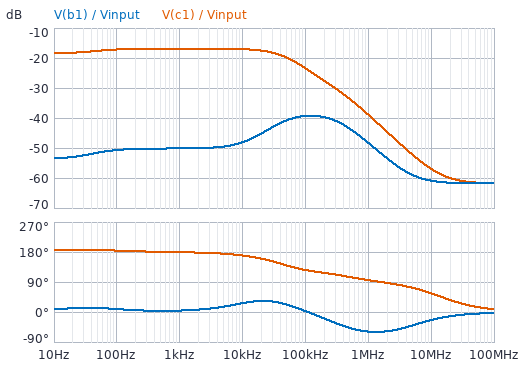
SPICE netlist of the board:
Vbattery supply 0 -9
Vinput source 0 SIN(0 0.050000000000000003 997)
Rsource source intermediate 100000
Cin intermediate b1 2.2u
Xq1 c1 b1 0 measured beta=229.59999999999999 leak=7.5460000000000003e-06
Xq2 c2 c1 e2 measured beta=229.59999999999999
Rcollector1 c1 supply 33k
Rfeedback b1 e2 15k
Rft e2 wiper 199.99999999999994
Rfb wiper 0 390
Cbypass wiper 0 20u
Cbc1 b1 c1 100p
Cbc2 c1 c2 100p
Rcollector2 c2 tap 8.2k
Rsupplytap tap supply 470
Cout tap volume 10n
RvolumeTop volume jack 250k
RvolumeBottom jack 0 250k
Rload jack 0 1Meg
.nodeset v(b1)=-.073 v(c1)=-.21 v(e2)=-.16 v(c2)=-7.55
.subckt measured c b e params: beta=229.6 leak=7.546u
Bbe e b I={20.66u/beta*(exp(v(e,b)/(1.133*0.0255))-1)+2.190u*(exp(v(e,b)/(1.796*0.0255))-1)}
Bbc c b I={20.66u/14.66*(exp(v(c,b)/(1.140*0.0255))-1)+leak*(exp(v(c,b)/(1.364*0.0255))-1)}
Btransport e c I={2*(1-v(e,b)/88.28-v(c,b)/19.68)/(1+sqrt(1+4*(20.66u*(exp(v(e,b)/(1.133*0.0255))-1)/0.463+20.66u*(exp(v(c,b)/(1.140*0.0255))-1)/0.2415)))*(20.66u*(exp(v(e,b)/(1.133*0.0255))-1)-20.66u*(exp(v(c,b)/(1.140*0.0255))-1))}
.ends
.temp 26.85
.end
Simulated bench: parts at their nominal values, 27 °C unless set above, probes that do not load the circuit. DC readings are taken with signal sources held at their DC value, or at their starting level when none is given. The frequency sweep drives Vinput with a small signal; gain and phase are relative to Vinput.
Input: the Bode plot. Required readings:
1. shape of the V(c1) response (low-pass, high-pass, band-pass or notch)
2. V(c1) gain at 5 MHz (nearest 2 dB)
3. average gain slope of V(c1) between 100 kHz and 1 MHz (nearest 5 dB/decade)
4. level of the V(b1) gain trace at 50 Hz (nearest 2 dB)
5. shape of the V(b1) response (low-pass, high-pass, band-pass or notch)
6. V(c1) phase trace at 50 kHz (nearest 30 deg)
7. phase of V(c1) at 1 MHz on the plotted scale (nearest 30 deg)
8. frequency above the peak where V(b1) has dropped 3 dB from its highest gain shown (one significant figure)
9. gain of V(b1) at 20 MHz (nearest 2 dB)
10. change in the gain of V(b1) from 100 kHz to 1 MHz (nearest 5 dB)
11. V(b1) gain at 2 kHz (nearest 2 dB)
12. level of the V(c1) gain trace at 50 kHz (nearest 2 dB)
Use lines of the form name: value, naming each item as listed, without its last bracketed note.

shape of the V(c1) response: low-pass
V(c1) gain at 5 MHz: -52 dB
average gain slope of V(c1) between 100 kHz and 1 MHz: -15 dB/decade
level of the V(b1) gain trace at 50 Hz: -52 dB
shape of the V(b1) response: band-pass
V(c1) phase trace at 50 kHz: 150 deg
phase of V(c1) at 1 MHz on the plotted scale: 90 deg
frequency above the peak where V(b1) has dropped 3 dB from its highest gain shown: 400 kHz
gain of V(b1) at 20 MHz: -62 dB
change in the gain of V(b1) from 100 kHz to 1 MHz: -10 dB
V(b1) gain at 2 kHz: -50 dB
level of the V(c1) gain trace at 50 kHz: -20 dB
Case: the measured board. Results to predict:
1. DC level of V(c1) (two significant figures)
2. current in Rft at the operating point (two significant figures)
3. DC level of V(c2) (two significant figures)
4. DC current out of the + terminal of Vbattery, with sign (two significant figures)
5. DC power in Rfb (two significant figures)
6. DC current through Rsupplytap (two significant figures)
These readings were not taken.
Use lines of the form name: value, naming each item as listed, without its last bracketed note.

DC level of V(c1): -150 mV
current in Rft at the operating point: 170 µA
DC level of V(c2): -7.5 V
DC current out of the + terminal of Vbattery, with sign: -440 µA
DC power in Rfb: 11 µW
DC current through Rsupplytap: 180 µA
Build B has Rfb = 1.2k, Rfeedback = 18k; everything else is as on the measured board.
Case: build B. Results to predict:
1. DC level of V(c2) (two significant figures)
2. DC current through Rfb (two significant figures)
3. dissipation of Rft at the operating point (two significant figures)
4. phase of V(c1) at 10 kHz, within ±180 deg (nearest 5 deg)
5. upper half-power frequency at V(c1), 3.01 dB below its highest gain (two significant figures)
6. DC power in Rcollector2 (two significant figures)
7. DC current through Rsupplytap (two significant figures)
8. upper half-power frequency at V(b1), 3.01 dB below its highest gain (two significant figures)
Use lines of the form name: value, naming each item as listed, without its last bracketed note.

DC level of V(c2): -8.2 V
DC current through Rfb: 81 µA
dissipation of Rft at the operating point: 1.3 µW
phase of V(c1) at 10 kHz, within ±180 deg: 170 deg
upper half-power frequency at V(c1), 3.01 dB below its highest gain: 55 kHz
DC power in Rcollector2: 66 µW
DC current through Rsupplytap: 90 µA
upper half-power frequency at V(b1), 3.01 dB below its highest gain: 370 kHz
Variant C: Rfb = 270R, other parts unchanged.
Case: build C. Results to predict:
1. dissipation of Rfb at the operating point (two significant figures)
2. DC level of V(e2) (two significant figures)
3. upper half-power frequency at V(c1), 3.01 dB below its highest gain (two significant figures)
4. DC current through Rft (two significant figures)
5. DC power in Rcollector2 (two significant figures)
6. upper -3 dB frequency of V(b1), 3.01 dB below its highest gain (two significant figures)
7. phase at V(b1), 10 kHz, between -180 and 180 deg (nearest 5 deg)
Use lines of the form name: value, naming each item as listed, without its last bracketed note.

dissipation of Rfb at the operating point: 12 µW
DC level of V(e2): -98 mV
upper half-power frequency at V(c1), 3.01 dB below its highest gain: 49 kHz
DC current through Rft: 210 µA
DC power in Rcollector2: 370 µW
upper -3 dB frequency of V(b1), 3.01 dB below its highest gain: 410 kHz
phase at V(b1), 10 kHz, between -180 and 180 deg: 30 deg
